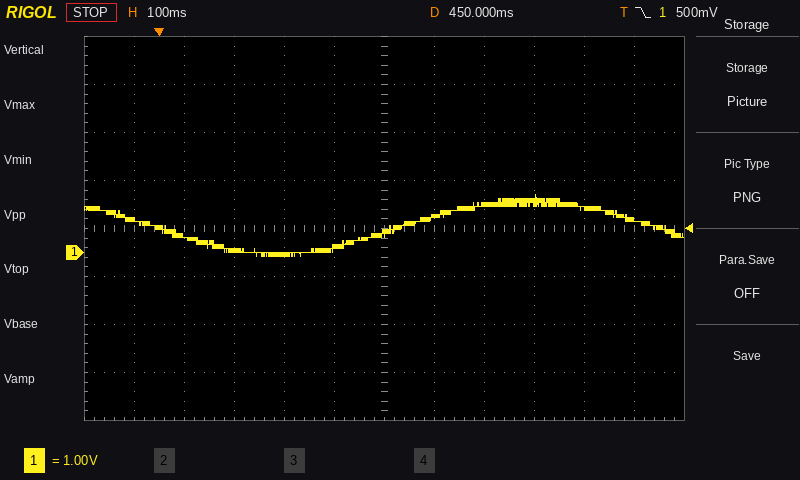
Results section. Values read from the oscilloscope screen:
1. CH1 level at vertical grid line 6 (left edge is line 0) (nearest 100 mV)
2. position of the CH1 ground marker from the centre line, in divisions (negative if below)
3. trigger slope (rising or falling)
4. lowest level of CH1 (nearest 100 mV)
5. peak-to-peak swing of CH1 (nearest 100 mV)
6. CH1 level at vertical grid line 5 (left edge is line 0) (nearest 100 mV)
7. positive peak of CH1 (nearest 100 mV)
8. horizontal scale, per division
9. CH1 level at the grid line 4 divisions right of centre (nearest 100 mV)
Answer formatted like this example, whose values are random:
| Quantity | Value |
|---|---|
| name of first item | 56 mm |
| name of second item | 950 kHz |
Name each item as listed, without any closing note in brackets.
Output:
| Quantity | Value |
|---|---|
| CH1 level at vertical grid line 6 (left edge is line 0) | 400 mV |
| position of the CH1 ground marker from the centre line, in divisions | -0.5 div |
| trigger slope | falling |
| lowest level of CH1 | -100 mV |
| peak-to-peak swing of CH1 | 1.3 V |
| CH1 level at vertical grid line 5 (left edge is line 0) | 100 mV |
| positive peak of CH1 | 1.2 V |
| horizontal scale, per division | 100 ms |
| CH1 level at the grid line 4 divisions right of centre | 900 mV |
